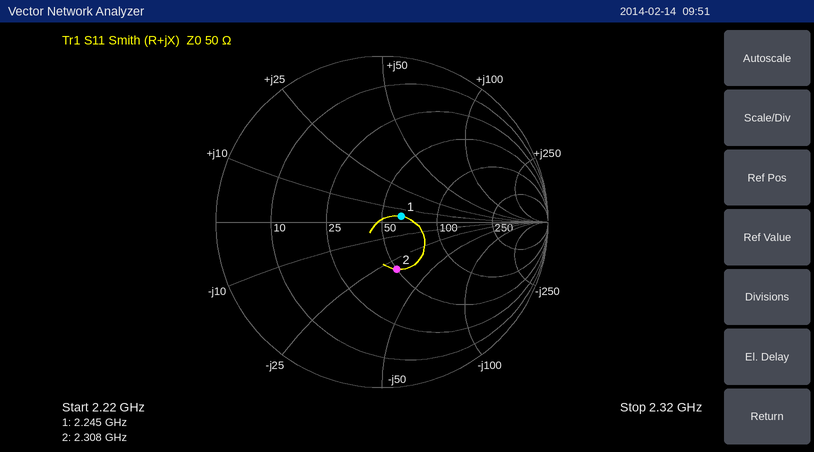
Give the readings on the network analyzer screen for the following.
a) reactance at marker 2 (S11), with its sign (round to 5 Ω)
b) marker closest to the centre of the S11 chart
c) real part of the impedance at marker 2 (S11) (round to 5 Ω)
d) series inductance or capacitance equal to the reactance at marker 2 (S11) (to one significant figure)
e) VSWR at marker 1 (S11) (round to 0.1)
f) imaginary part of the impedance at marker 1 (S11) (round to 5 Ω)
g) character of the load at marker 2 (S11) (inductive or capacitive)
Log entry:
-30 Ω
marker 1
50 Ω
2 pF
1.3
+5 Ω
capacitive
